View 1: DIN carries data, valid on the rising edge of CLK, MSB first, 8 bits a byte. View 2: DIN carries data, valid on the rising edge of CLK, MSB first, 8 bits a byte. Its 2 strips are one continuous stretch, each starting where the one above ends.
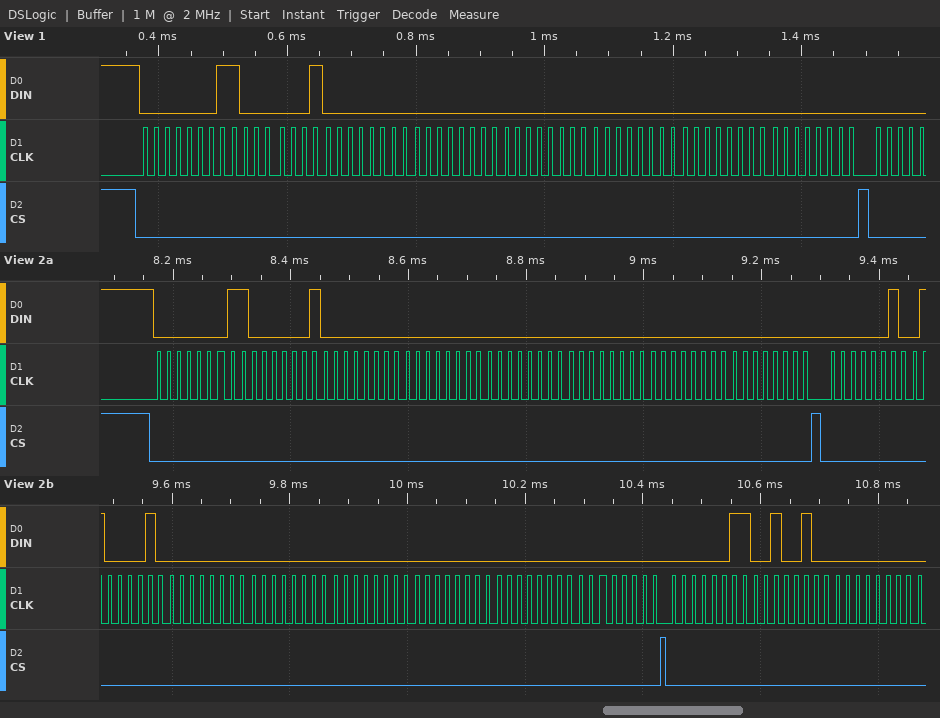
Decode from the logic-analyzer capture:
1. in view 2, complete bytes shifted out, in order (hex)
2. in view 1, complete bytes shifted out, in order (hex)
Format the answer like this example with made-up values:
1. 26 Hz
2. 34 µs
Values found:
1. 01 81 00 00 00 00 00 00 02 42 00 00 00 00 00 00 03 24 00
2. 0x01 0x81 0x00 0x00 0x00 0x00 0x00 0x00
